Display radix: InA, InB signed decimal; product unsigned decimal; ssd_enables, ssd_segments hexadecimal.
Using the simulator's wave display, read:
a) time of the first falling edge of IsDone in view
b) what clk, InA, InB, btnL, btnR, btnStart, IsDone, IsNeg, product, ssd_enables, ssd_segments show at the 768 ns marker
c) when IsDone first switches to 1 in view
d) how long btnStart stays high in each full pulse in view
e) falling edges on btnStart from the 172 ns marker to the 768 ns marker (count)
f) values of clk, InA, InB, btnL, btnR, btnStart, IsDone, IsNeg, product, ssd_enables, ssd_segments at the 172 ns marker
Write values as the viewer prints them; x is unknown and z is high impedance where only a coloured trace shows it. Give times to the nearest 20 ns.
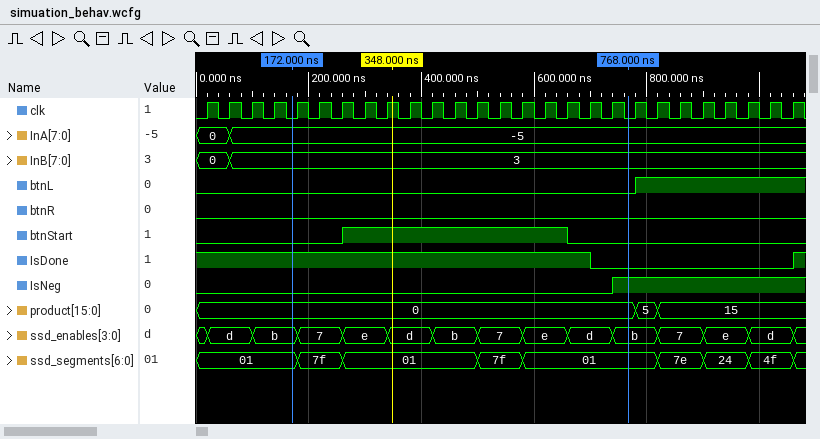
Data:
700 ns
clk=0, InA=-5, InB=3, btnL=0, btnR=0, btnStart=0, IsDone=0, IsNeg=1, product=0, ssd_enables=b, ssd_segments=01
1060 ns
400 ns
1
clk=0, InA=-5, InB=3, btnL=0, btnR=0, btnStart=0, IsDone=1, IsNeg=0, product=0, ssd_enables=b, ssd_segments=01
